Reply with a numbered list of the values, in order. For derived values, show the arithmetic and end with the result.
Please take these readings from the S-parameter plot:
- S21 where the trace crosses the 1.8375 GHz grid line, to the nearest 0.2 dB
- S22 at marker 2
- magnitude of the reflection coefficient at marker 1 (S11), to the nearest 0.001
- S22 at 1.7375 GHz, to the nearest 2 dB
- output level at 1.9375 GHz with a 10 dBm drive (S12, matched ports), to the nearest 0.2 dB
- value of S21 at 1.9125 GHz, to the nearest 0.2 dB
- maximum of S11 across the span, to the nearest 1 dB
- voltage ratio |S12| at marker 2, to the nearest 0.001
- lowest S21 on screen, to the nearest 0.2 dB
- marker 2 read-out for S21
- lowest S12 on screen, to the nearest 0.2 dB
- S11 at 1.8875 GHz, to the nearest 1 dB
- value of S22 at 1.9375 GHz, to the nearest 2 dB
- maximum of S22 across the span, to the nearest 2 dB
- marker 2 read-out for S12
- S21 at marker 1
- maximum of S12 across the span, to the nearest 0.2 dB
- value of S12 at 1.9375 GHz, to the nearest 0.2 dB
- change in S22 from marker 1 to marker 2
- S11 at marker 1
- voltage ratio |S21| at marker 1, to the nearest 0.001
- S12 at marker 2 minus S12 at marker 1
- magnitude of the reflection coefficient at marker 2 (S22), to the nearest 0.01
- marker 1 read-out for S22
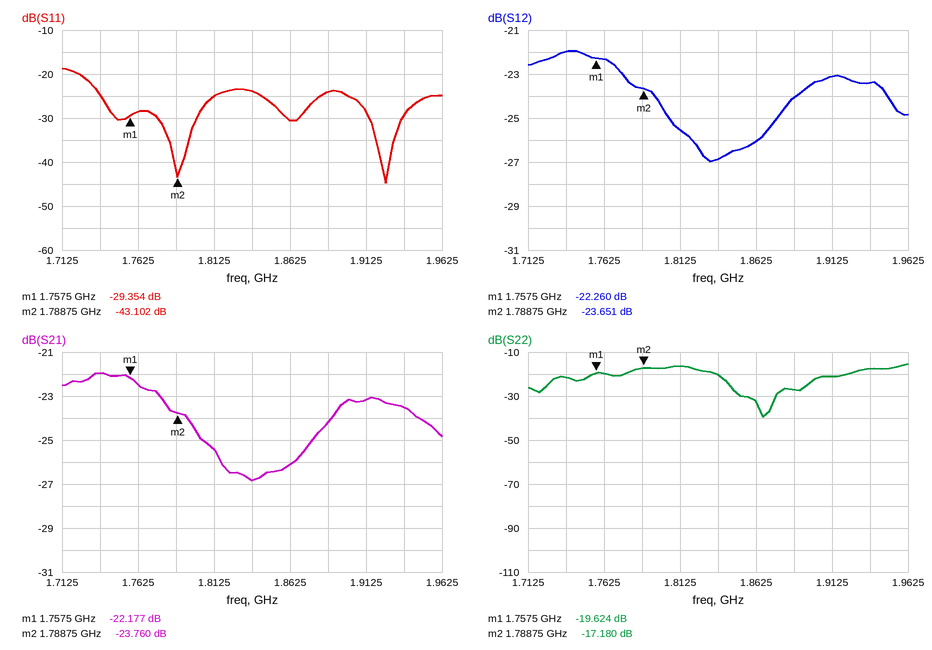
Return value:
1. -26.8 dB
2. -17.180 dB
3. 10^(-29.354/20) ≈ 0.034
4. -22 dB
5. 10 dBm + (-23.4 dB) = -13.4 dBm
6. -23.2 dB
7. -19 dB
8. 10^(-23.651/20) ≈ 0.066
9. -26.8 dB
10. -23.760 dB
11. -27.0 dB
12. -24 dB
13. -18 dB
14. -16 dB
15. -23.651 dB
16. -22.177 dB
17. -22.0 dB
18. -23.4 dB
19. -17.18 − (-19.624) = 2.444 dB
20. -29.354 dB
21. 10^(-22.177/20) ≈ 0.078
22. -23.651 − (-22.26) = -1.391 dB
23. 10^(-17.18/20) ≈ 0.14
24. -19.624 dB
